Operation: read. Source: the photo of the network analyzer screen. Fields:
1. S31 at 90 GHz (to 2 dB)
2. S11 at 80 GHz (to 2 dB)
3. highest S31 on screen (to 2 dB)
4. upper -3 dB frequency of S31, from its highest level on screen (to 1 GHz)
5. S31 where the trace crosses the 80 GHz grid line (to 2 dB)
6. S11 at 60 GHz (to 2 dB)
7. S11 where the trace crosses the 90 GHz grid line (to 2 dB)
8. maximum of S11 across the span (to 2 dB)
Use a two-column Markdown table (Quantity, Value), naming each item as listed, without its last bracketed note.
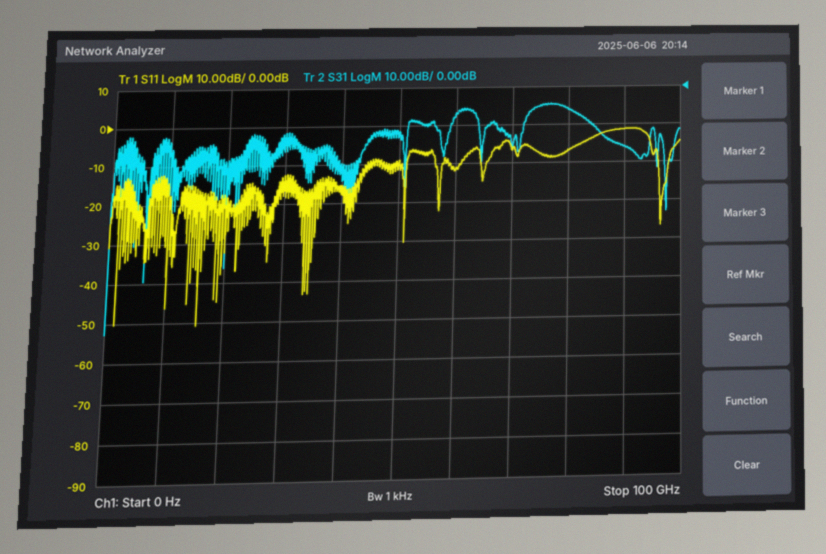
| Quantity | Value |
|---|---|
| S31 at 90 GHz | -16 dB |
| S11 at 80 GHz | -6 dB |
| highest S31 on screen | -4 dB |
| upper -3 dB frequency of S31, from its highest level on screen | 82 GHz |
| S31 where the trace crosses the 80 GHz grid line | -6 dB |
| S11 at 60 GHz | -12 dB |
| S11 where the trace crosses the 90 GHz grid line | -2 dB |
| maximum of S11 across the span | -2 dB |
